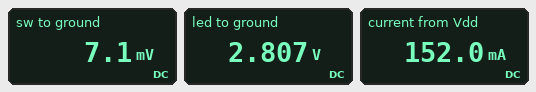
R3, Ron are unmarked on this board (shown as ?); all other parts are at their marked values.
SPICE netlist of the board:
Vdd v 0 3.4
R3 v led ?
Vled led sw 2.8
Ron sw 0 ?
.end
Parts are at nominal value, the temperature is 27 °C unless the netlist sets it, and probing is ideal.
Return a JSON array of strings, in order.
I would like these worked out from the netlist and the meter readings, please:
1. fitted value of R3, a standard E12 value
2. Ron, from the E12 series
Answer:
["3.9 Ω", "0.047 Ω"]
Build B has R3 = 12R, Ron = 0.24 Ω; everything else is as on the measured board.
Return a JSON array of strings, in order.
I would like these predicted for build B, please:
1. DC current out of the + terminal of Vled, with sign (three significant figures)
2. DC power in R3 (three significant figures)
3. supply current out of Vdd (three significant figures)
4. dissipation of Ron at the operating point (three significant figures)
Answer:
["-49.0 mA", "28.8 mW", "49.0 mA", "577 µW"]
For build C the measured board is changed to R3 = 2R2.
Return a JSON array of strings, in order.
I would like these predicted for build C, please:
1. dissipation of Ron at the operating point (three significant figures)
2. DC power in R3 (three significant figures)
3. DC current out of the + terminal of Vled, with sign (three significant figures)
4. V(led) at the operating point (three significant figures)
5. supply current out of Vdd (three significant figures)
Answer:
["3.35 mW", "157 mW", "-267 mA", "2.81 V", "267 mA"]
